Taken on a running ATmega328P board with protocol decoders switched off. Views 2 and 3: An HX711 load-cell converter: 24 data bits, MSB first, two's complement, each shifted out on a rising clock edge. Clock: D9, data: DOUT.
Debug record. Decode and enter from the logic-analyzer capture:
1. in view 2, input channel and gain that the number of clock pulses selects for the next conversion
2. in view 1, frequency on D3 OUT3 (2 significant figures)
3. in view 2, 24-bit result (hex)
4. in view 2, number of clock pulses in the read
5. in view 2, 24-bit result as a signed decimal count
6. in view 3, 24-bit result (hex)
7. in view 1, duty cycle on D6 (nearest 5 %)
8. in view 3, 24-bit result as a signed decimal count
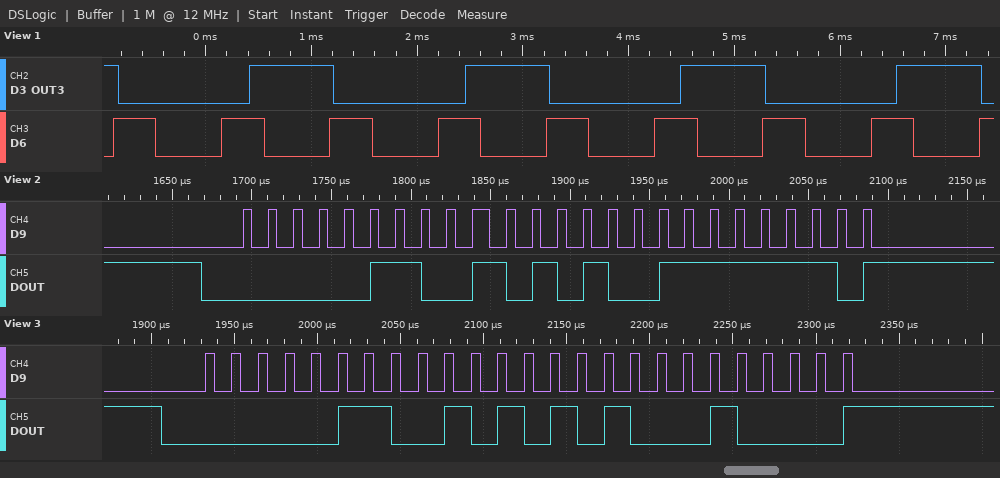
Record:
channel A, gain 128
490 Hz
0x0654FE
25
414974
0x065510
40 %
414992
